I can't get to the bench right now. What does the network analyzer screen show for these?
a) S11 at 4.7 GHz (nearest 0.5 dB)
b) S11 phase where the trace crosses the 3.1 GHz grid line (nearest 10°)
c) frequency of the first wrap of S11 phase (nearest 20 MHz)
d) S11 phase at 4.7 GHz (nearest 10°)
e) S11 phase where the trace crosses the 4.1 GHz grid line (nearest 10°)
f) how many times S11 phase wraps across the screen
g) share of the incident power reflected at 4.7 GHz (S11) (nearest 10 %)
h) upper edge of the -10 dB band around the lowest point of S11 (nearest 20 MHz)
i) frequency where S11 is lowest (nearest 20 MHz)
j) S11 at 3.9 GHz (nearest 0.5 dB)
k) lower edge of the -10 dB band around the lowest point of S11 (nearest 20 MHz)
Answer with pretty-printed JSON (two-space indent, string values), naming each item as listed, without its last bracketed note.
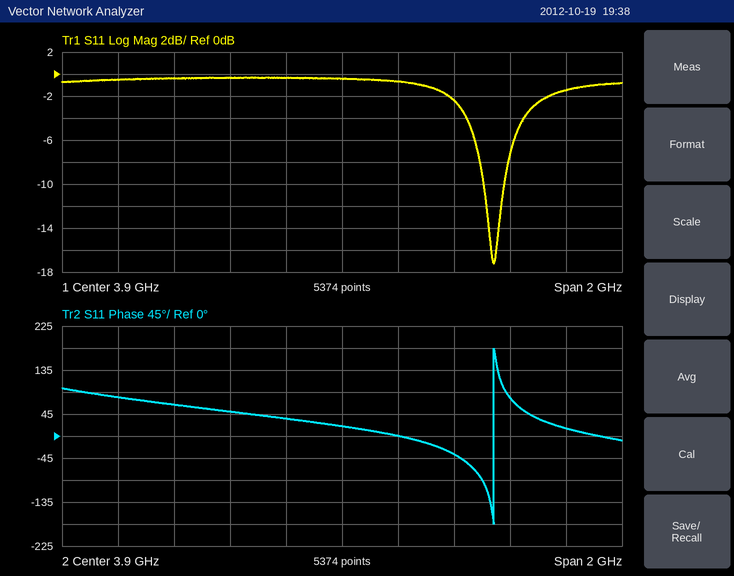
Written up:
{
  "S11 at 4.7 GHz": "-1.5 dB",
  "S11 phase where the trace crosses the 3.1 GHz grid line": "80°",
  "frequency of the first wrap of S11 phase": "4.44 GHz",
  "S11 phase at 4.7 GHz": "20°",
  "S11 phase where the trace crosses the 4.1 GHz grid line": "0°",
  "how many times S11 phase wraps across the screen": "1",
  "share of the incident power reflected at 4.7 GHz (S11)": "70 %",
  "upper edge of the -10 dB band around the lowest point of S11": "4.48 GHz",
  "frequency where S11 is lowest": "4.44 GHz",
  "S11 at 3.9 GHz": "-0.5 dB",
  "lower edge of the -10 dB band around the lowest point of S11": "4.40 GHz"
}
